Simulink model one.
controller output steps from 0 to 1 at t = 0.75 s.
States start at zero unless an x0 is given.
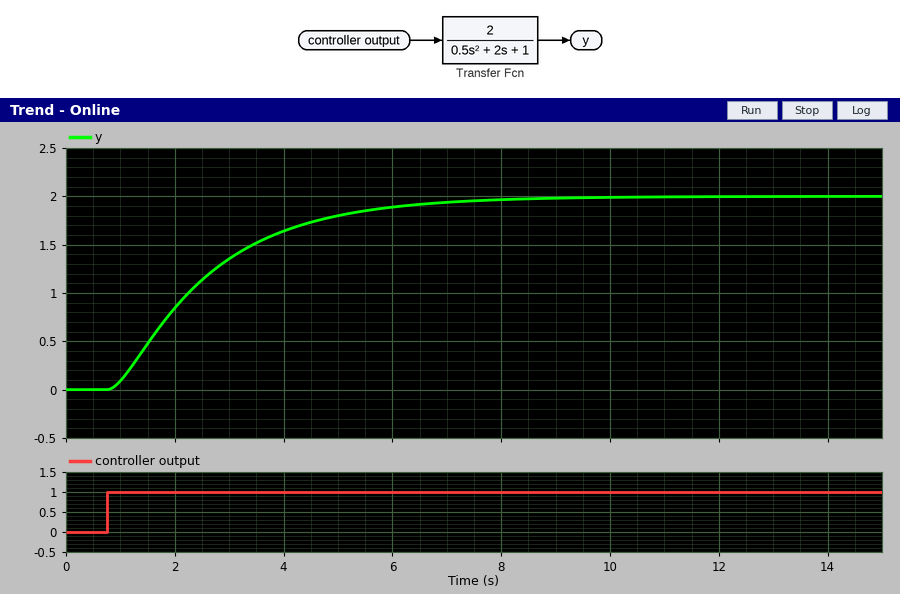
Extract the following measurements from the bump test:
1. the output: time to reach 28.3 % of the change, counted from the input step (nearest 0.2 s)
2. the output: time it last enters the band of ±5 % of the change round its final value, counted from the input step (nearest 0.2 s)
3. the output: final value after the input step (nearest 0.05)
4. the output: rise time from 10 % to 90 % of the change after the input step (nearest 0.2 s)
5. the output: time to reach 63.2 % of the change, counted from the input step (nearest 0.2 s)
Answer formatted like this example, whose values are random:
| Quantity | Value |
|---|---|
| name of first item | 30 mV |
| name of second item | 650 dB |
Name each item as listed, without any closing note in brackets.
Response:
| Quantity | Value |
|---|---|
| the output: time to reach 28.3 % of the change, counted from the input step | 0.8 s |
| the output: time it last enters the band of ±5 % of the change round its final value, counted from the input step | 5.4 s |
| the output: final value after the input step | 2.00 |
| the output: rise time from 10 % to 90 % of the change after the input step | 3.8 s |
| the output: time to reach 63.2 % of the change, counted from the input step | 2.0 s |
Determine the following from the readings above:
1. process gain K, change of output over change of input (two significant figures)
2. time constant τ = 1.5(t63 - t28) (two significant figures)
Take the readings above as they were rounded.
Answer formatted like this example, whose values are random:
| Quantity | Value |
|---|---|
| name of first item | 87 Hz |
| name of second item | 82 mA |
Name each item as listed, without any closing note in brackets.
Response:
| Quantity | Value |
|---|---|
| process gain K, change of output over change of input | 2.0 |
| time constant τ = 1.5(t63 - t28) | 1.8 s |
